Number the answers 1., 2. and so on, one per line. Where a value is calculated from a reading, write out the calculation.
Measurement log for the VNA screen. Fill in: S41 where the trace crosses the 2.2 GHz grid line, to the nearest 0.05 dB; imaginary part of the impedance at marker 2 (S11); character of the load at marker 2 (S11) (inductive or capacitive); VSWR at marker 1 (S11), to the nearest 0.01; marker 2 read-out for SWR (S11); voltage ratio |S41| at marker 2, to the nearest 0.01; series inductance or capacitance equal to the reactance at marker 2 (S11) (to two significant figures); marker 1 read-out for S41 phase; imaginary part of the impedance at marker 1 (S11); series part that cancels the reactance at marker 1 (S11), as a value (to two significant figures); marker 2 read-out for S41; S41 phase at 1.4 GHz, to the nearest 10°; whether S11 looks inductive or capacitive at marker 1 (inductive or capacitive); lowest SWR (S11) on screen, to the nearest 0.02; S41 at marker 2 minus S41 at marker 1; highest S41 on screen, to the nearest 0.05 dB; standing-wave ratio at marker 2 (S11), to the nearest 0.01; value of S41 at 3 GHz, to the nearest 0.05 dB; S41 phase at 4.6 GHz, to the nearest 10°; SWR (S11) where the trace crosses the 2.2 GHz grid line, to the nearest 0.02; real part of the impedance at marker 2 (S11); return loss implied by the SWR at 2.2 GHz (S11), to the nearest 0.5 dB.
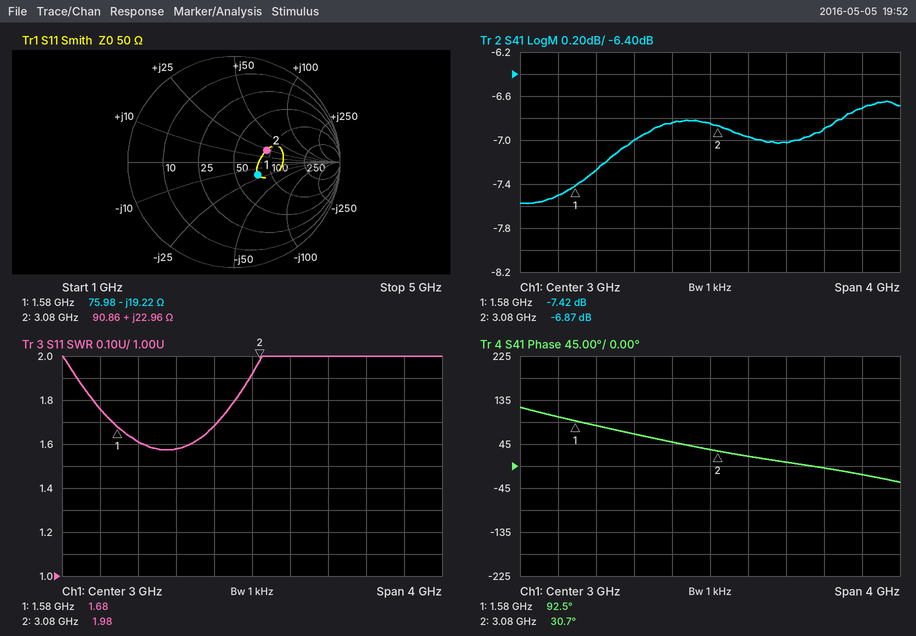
1. -7.00 dB
2. +22.96 Ω
3. inductive
4. 1.68
5. 1.98
6. 10^(-6.87/20) ≈ 0.45
7. L = 22.96 Ω/(2π × 3.08 GHz) ≈ 1.2 nH
8. 92.5°
9. -19.22 Ω
10. L = 19.22 Ω/(2π × 1.58 GHz) ≈ 1.9 nH
11. -6.87 dB
12. 100°
13. capacitive
14. 1.58
15. -6.87 − (-7.42) = 0.55 dB
16. -6.65 dB
17. 1.98
18. -6.85 dB
19. -20°
20. 1.58
21. 90.86 Ω
22. −20 log10((1.58 − 1)/(1.58 + 1)) ≈ 13.0 dB
